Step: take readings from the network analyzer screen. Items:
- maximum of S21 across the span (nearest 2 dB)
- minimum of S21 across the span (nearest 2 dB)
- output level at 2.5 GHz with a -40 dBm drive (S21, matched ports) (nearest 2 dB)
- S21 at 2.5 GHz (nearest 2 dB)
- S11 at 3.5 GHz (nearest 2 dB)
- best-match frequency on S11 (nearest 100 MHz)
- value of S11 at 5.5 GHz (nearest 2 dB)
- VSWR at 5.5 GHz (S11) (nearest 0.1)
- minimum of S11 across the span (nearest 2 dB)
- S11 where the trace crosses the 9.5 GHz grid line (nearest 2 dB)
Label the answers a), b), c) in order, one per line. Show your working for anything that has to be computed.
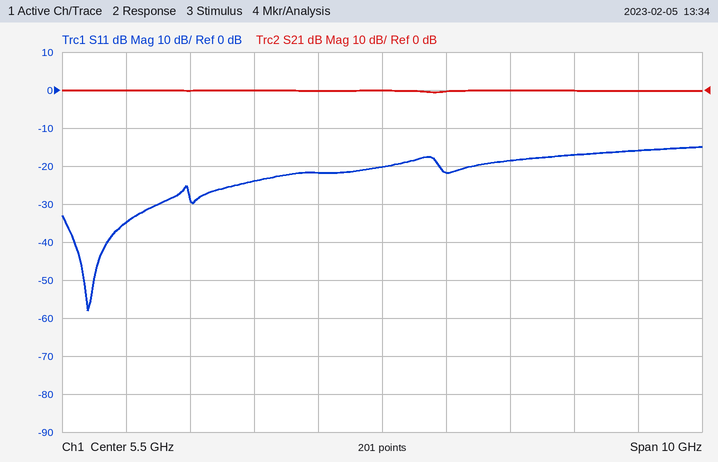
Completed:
a) 0 dB
b) 0 dB
c) -40 dBm + (0 dB) = -40 dBm
d) 0 dB
e) -24 dB
f) 900 MHz
g) -20 dB
h) |Γ| = 10^(-20/20) = 0.1000; VSWR = (1 + 0.1000)/(1 − 0.1000) ≈ 1.2
i) -58 dB
j) -16 dB
